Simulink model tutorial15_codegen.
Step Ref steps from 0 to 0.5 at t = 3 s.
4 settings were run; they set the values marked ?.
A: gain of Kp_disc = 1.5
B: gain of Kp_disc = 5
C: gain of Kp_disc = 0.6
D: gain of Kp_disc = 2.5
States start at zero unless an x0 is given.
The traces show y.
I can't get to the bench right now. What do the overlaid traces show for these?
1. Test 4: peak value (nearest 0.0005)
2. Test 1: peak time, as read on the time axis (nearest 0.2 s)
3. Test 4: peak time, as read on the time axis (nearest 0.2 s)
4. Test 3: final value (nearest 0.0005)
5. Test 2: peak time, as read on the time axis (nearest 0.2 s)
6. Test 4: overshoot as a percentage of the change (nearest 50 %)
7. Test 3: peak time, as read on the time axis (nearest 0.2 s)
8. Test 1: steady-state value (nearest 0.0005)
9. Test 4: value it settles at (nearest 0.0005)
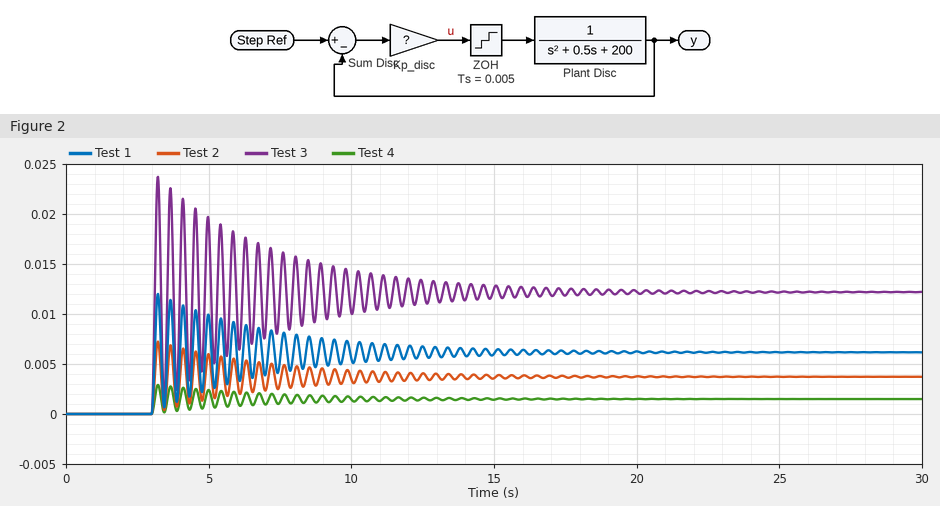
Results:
0.0030
3.2 s
3.2 s
0.0120
3.2 s
100 %
3.2 s
0.0060
0.0015
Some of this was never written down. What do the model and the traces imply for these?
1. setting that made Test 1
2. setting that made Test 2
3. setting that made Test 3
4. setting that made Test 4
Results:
D
A
B
C
